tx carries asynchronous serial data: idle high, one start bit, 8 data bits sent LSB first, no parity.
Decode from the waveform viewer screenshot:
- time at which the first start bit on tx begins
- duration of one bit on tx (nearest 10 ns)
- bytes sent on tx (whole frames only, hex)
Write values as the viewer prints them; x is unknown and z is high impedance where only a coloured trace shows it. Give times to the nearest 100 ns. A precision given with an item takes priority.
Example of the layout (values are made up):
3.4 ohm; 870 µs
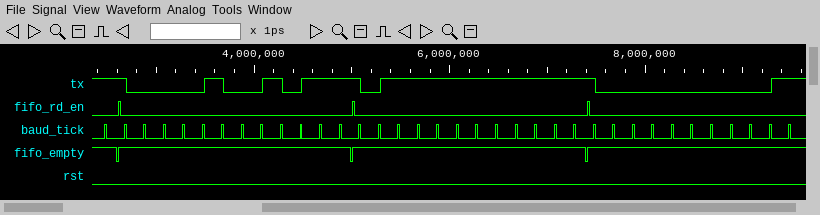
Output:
2700 ns; 200 ns; 48, FF, 00
